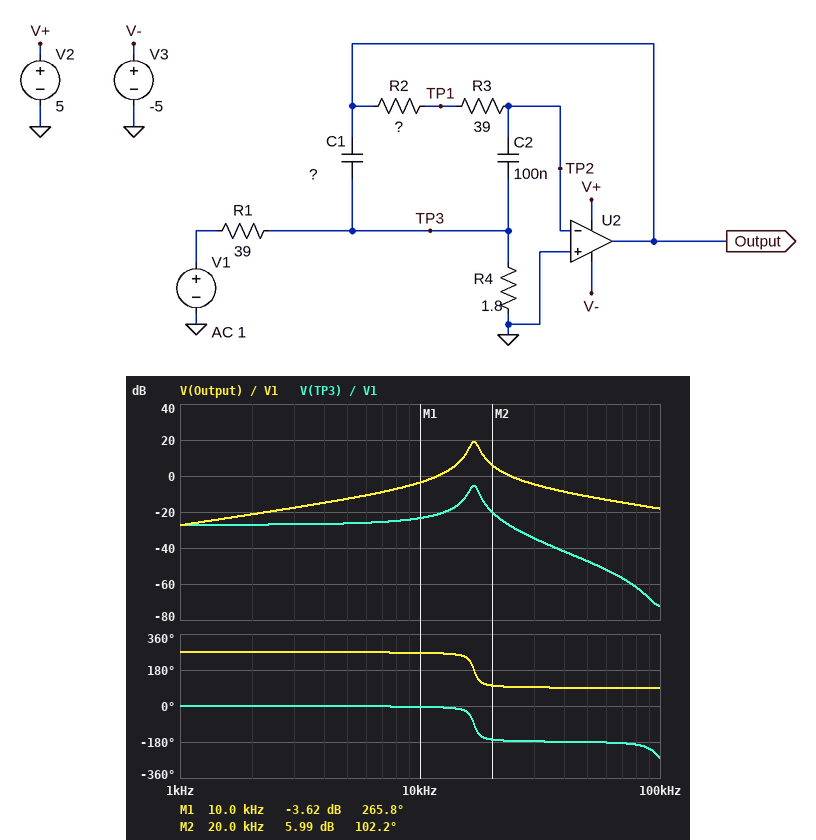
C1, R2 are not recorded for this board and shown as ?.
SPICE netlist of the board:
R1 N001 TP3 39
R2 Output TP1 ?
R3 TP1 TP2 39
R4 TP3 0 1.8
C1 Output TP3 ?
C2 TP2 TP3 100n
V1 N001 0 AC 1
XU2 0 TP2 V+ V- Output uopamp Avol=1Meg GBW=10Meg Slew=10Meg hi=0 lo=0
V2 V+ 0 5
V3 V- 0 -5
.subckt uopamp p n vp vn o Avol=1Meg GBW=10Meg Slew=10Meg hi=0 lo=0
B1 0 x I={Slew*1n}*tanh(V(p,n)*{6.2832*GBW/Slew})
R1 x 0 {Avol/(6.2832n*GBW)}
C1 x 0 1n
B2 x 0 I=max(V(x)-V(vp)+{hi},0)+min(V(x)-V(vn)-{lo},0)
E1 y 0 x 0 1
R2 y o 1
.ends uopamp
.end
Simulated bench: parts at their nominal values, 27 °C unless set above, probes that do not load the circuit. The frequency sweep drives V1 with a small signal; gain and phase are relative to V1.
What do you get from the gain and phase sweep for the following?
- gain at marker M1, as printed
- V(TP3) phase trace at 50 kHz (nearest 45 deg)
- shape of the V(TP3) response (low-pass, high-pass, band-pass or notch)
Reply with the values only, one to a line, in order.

-3.62 dB
-180 deg
low-pass
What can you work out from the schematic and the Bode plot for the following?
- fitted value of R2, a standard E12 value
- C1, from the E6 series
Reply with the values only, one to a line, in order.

1.5 kΩ
330 nF
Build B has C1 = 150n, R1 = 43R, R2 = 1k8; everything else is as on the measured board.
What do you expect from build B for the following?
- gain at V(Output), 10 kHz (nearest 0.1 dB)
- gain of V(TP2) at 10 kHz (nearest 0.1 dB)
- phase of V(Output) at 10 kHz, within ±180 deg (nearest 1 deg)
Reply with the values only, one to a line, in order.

-4.7 dB
-64.7 dB
-92 deg
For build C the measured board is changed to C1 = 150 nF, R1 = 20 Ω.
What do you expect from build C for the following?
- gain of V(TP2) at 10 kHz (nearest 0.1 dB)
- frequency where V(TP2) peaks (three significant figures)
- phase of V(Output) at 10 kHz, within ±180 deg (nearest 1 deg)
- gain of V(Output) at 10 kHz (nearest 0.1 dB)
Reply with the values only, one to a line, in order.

-60.4 dB
25.0 kHz
-92 deg
-0.4 dB
